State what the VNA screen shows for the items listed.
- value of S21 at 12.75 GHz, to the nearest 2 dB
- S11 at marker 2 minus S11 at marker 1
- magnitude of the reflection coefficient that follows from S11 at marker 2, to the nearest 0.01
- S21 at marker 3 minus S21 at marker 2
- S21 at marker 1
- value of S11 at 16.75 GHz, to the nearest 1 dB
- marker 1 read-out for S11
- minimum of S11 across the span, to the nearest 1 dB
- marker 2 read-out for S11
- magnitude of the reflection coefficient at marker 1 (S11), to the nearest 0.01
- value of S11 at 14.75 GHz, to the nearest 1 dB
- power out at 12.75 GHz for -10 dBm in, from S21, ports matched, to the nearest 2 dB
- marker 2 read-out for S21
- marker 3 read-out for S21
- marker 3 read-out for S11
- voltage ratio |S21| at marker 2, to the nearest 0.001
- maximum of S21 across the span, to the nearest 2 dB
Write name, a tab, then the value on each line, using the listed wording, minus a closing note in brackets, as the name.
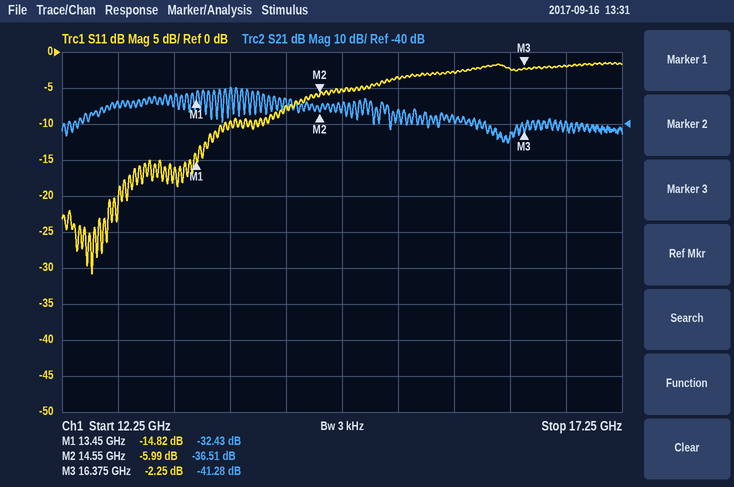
value of S21 at 12.75 GHz, to the nearest 2 dB	-34 dB
S11 at marker 2 minus S11 at marker 1	8.83 dB
magnitude of the reflection coefficient that follows from S11 at marker 2, to the nearest 0.01	0.50
S21 at marker 3 minus S21 at marker 2	-4.77 dB
S21 at marker 1	-32.43 dB
value of S11 at 16.75 GHz, to the nearest 1 dB	-2 dB
marker 1 read-out for S11	-14.82 dB
minimum of S11 across the span, to the nearest 1 dB	-31 dB
marker 2 read-out for S11	-5.99 dB
magnitude of the reflection coefficient at marker 1 (S11), to the nearest 0.01	0.18
value of S11 at 14.75 GHz, to the nearest 1 dB	-5 dB
power out at 12.75 GHz for -10 dBm in, from S21, ports matched, to the nearest 2 dB	-44 dBm
marker 2 read-out for S21	-36.51 dB
marker 3 read-out for S21	-41.28 dB
marker 3 read-out for S11	-2.25 dB
voltage ratio |S21| at marker 2, to the nearest 0.001	0.015
maximum of S21 across the span, to the nearest 2 dB	-30 dB
